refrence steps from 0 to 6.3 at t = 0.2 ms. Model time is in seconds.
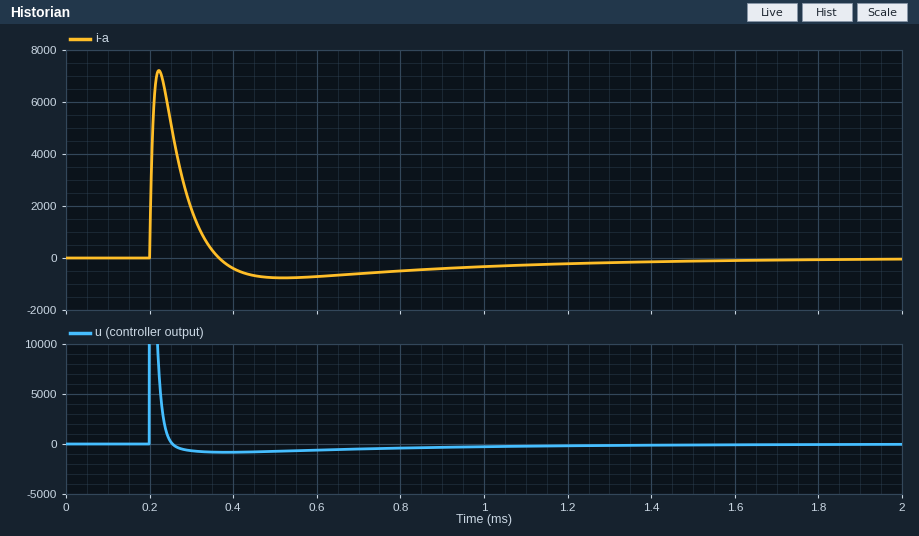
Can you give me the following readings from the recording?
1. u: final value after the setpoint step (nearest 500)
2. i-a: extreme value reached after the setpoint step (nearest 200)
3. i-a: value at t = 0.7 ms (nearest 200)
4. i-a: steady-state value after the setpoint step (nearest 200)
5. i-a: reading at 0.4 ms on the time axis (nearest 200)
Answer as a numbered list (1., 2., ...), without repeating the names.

1. 0
2. 7200
3. -600
4. 0
5. -400
